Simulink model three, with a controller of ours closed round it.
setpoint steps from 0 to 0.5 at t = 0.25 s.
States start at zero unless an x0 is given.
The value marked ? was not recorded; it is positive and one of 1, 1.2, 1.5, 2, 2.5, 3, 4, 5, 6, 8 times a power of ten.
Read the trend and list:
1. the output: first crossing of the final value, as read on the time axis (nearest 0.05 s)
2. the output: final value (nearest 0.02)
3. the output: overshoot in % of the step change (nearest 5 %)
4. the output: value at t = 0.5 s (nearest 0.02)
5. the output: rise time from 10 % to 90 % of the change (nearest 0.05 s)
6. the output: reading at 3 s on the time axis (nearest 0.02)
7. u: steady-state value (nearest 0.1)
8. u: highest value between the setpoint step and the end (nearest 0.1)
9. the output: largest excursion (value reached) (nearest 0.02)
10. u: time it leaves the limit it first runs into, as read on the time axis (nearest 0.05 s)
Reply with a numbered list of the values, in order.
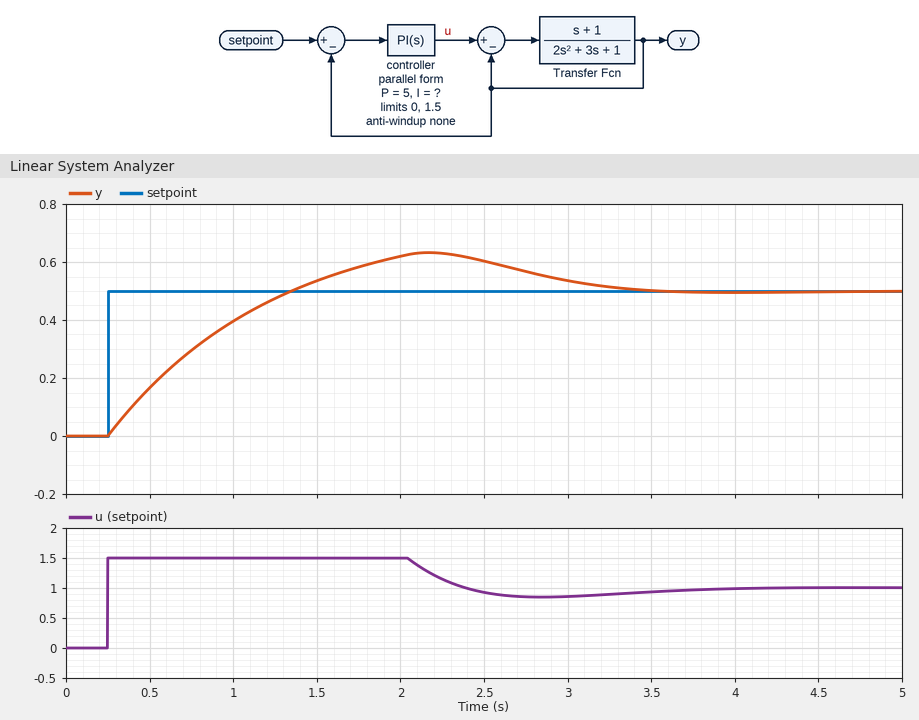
1. 1.35 s
2. 0.50
3. 25 %
4. 0.16
5. 0.85 s
6. 0.54
7. 1.0
8. 1.5
9. 0.64
10. 2.05 s
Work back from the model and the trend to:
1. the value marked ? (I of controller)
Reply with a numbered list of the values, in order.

1. 12
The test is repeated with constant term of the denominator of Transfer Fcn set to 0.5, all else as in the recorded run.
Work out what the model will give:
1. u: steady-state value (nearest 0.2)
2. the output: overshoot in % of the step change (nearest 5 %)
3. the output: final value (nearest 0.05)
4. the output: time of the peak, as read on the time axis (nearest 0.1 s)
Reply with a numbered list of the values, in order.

1. 0.8
2. 30 %
3. 0.50
4. 2.0 s
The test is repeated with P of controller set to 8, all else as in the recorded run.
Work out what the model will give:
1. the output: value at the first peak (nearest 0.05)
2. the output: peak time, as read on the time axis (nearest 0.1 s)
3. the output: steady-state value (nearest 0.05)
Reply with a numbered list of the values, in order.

1. 0.60
2. 2.0 s
3. 0.50
